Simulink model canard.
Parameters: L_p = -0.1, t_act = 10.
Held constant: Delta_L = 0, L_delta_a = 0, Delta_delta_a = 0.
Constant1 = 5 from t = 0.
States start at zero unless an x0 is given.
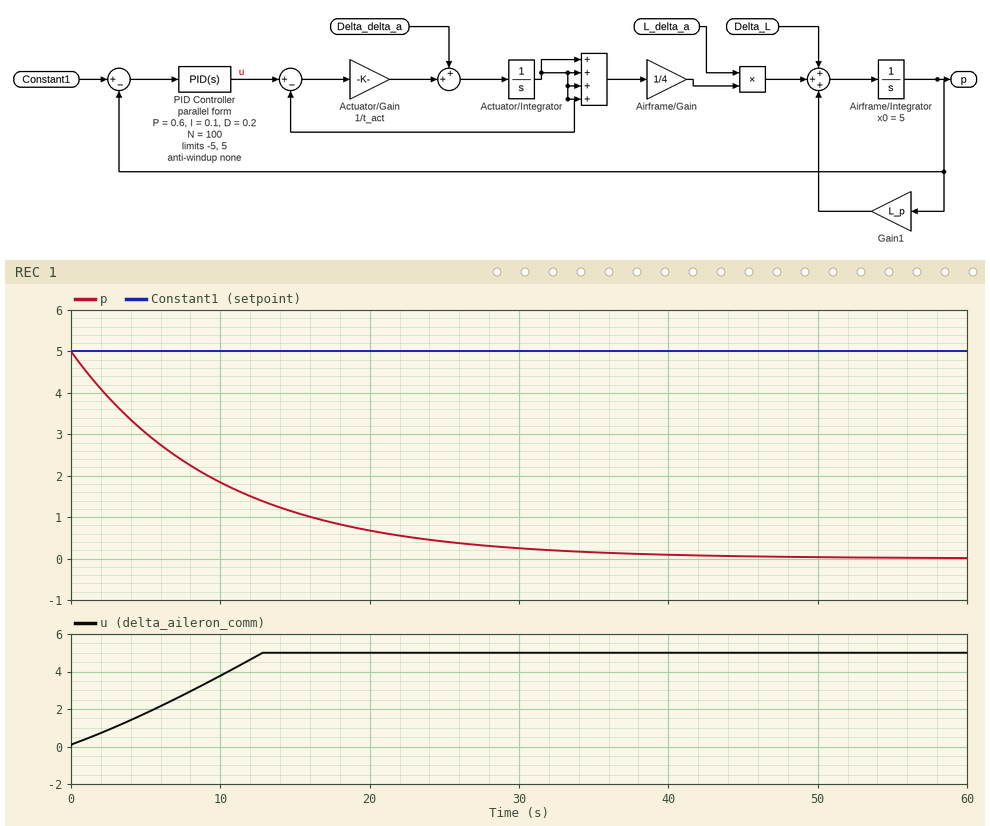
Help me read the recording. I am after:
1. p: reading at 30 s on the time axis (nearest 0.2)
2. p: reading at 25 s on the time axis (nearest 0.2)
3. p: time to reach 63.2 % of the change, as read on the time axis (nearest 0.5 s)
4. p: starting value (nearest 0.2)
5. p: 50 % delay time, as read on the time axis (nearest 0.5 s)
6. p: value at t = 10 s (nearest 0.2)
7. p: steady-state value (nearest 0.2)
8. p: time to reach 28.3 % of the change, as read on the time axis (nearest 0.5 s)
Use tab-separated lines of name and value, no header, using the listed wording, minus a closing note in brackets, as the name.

p: reading at 30 s on the time axis	0.2
p: reading at 25 s on the time axis	0.4
p: time to reach 63.2 % of the change, as read on the time axis	10.0 s
p: starting value	5.0
p: 50 % delay time, as read on the time axis	7.0 s
p: value at t = 10 s	1.8
p: steady-state value	0.0
p: time to reach 28.3 % of the change, as read on the time axis	3.5 s
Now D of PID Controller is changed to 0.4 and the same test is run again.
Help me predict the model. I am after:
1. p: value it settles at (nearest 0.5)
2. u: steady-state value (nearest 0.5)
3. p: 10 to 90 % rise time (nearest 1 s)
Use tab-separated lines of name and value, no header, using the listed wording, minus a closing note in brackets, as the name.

p: value it settles at	0.0
u: steady-state value	5.0
p: 10 to 90 % rise time	22 s
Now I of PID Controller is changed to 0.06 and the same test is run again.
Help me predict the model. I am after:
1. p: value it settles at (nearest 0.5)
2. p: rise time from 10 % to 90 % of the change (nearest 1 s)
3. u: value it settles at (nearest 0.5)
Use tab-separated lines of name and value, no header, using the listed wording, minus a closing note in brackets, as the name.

p: value it settles at	0.0
p: rise time from 10 % to 90 % of the change	22 s
u: value it settles at	5.0
